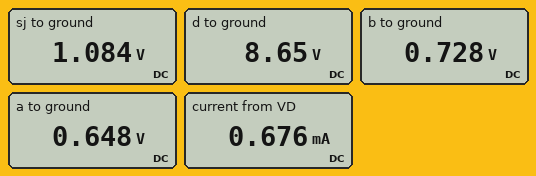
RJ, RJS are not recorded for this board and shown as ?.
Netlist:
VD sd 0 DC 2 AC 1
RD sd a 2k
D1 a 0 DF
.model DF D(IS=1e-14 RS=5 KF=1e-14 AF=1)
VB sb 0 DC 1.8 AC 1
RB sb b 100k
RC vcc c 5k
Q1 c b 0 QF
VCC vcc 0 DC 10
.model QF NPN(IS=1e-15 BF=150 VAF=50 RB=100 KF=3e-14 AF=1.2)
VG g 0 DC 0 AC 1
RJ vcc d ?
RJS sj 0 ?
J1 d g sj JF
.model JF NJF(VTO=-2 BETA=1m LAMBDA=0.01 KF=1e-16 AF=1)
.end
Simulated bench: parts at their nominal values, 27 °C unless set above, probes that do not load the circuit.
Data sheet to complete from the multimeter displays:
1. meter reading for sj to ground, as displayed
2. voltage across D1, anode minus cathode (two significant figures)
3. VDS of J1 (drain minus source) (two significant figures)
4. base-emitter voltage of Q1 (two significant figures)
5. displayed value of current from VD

1.084 V
650 mV
7.6 V
730 mV
0.676 mA
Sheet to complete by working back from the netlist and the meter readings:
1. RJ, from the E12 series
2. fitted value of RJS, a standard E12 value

1.5 kΩ
1.2 kΩ
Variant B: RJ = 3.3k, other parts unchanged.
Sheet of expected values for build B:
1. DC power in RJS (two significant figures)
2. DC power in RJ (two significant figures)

970 µW
2.7 mW
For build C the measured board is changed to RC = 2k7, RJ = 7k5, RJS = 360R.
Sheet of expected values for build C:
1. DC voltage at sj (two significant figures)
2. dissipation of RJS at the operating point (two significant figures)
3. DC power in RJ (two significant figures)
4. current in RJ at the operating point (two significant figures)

440 mV
530 µW
11 mW
1.2 mA
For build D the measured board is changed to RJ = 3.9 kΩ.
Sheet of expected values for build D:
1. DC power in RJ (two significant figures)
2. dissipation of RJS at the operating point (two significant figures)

3.1 mW
970 µW
